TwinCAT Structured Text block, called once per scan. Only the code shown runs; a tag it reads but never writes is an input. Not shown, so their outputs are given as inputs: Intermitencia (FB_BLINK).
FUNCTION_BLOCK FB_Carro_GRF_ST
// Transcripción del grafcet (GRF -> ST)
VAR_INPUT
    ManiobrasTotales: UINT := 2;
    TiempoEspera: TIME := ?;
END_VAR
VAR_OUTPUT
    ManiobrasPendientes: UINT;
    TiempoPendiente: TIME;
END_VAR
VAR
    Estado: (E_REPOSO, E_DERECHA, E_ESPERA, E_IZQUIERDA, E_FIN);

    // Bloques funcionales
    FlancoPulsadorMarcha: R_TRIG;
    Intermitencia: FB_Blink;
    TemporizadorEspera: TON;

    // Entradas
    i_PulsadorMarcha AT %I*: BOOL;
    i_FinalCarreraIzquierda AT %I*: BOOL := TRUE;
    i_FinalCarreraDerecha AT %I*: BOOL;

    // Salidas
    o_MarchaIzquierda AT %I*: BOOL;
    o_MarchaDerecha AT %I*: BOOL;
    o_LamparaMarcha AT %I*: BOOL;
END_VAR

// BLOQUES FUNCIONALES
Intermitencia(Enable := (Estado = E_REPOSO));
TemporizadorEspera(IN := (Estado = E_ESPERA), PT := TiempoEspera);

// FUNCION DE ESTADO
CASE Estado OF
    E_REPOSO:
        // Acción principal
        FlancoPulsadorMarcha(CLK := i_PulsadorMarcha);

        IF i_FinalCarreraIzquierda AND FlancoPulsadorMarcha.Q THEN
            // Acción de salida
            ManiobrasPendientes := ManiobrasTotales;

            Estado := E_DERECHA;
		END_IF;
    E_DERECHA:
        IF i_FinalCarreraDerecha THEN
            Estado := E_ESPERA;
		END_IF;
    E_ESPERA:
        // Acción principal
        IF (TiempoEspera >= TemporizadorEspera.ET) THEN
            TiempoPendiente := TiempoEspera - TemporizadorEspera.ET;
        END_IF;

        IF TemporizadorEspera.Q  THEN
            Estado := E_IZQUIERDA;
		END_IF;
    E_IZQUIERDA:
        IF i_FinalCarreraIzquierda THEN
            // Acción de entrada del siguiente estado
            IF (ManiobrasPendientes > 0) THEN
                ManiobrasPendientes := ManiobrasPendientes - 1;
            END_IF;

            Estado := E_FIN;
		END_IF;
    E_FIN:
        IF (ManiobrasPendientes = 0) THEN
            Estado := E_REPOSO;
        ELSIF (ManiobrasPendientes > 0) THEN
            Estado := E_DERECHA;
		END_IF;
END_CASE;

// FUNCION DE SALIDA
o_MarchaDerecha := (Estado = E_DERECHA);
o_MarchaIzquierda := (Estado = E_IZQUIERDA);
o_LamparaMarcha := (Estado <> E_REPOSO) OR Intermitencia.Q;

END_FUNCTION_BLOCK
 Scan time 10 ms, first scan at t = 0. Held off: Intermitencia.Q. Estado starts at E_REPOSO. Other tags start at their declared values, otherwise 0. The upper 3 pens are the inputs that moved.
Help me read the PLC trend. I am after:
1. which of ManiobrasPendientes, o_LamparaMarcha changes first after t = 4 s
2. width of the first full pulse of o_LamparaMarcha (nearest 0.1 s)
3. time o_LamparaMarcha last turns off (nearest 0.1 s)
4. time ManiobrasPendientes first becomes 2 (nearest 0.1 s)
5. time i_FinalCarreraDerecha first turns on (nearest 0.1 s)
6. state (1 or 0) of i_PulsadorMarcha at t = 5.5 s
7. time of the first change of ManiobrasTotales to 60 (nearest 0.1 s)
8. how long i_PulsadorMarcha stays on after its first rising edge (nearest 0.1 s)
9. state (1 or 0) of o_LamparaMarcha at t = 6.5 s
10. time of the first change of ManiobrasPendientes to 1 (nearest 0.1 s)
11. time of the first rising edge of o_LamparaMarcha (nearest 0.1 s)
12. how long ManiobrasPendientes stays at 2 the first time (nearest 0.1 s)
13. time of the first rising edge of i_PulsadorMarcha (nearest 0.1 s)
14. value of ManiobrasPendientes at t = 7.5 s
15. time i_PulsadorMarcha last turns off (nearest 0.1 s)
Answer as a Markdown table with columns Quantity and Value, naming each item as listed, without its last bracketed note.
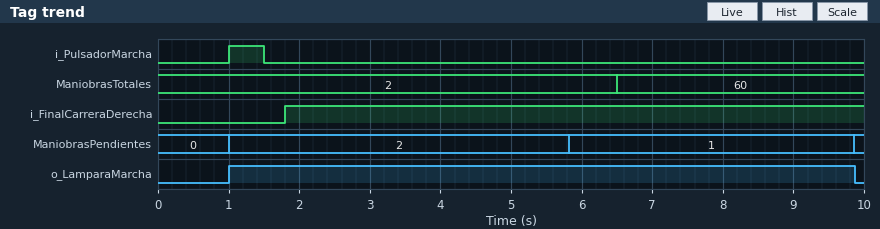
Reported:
| Quantity | Value |
|---|---|
| which of ManiobrasPendientes, o_LamparaMarcha changes first after t = 4 s | ManiobrasPendientes |
| width of the first full pulse of o_LamparaMarcha | 8.9 s |
| time o_LamparaMarcha last turns off | 9.9 s |
| time ManiobrasPendientes first becomes 2 | 1.0 s |
| time i_FinalCarreraDerecha first turns on | 1.8 s |
| state (1 or 0) of i_PulsadorMarcha at t = 5.5 s | 0 |
| time of the first change of ManiobrasTotales to 60 | 6.5 s |
| how long i_PulsadorMarcha stays on after its first rising edge | 0.5 s |
| state (1 or 0) of o_LamparaMarcha at t = 6.5 s | 1 |
| time of the first change of ManiobrasPendientes to 1 | 5.8 s |
| time of the first rising edge of o_LamparaMarcha | 1.0 s |
| how long ManiobrasPendientes stays at 2 the first time | 4.8 s |
| time of the first rising edge of i_PulsadorMarcha | 1.0 s |
| value of ManiobrasPendientes at t = 7.5 s | 1 |
| time i_PulsadorMarcha last turns off | 1.5 s |
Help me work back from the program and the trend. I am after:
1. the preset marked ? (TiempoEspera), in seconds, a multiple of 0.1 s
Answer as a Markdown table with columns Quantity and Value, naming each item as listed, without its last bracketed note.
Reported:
| Quantity | Value |
|---|---|
| the preset marked ? (TiempoEspera), in seconds, a multiple of 0.1 s | 4.0 s |
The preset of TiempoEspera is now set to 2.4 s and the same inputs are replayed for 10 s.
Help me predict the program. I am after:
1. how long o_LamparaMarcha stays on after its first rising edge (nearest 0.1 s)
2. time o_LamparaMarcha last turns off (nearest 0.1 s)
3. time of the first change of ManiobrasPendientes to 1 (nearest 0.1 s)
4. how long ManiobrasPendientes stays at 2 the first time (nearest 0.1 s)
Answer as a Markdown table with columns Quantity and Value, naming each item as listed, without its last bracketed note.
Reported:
| Quantity | Value |
|---|---|
| how long o_LamparaMarcha stays on after its first rising edge | 5.7 s |
| time o_LamparaMarcha last turns off | 6.7 s |
| time of the first change of ManiobrasPendientes to 1 | 4.2 s |
| how long ManiobrasPendientes stays at 2 the first time | 3.2 s |
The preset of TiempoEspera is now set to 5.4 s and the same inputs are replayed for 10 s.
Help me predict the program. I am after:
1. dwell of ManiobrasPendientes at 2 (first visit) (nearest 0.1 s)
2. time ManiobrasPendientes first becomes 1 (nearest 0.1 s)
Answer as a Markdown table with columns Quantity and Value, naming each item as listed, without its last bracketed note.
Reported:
| Quantity | Value |
|---|---|
| dwell of ManiobrasPendientes at 2 (first visit) | 6.2 s |
| time ManiobrasPendientes first becomes 1 | 7.2 s |
